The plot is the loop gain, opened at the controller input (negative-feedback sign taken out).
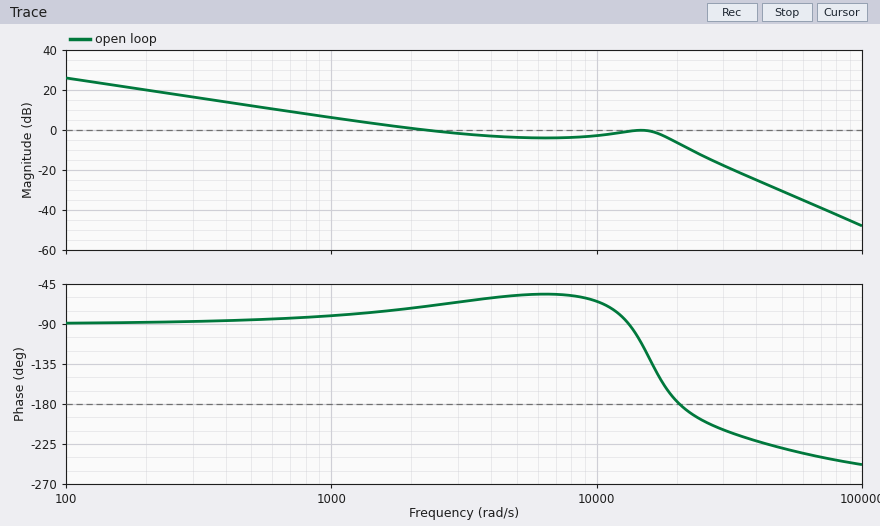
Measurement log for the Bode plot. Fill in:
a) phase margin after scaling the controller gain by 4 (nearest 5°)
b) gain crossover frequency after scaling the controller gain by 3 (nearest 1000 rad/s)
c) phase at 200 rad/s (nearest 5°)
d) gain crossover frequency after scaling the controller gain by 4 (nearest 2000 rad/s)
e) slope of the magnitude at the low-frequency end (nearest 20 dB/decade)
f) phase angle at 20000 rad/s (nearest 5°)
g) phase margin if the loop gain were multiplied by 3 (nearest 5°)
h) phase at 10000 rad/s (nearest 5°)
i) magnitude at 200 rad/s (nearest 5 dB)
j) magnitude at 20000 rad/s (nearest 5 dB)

-15°
22000 rad/s
-90°
24000 rad/s
-20 dB/decade
-175°
-10°
-65°
20 dB
-5 dB
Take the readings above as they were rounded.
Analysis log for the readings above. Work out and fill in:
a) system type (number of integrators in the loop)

1
